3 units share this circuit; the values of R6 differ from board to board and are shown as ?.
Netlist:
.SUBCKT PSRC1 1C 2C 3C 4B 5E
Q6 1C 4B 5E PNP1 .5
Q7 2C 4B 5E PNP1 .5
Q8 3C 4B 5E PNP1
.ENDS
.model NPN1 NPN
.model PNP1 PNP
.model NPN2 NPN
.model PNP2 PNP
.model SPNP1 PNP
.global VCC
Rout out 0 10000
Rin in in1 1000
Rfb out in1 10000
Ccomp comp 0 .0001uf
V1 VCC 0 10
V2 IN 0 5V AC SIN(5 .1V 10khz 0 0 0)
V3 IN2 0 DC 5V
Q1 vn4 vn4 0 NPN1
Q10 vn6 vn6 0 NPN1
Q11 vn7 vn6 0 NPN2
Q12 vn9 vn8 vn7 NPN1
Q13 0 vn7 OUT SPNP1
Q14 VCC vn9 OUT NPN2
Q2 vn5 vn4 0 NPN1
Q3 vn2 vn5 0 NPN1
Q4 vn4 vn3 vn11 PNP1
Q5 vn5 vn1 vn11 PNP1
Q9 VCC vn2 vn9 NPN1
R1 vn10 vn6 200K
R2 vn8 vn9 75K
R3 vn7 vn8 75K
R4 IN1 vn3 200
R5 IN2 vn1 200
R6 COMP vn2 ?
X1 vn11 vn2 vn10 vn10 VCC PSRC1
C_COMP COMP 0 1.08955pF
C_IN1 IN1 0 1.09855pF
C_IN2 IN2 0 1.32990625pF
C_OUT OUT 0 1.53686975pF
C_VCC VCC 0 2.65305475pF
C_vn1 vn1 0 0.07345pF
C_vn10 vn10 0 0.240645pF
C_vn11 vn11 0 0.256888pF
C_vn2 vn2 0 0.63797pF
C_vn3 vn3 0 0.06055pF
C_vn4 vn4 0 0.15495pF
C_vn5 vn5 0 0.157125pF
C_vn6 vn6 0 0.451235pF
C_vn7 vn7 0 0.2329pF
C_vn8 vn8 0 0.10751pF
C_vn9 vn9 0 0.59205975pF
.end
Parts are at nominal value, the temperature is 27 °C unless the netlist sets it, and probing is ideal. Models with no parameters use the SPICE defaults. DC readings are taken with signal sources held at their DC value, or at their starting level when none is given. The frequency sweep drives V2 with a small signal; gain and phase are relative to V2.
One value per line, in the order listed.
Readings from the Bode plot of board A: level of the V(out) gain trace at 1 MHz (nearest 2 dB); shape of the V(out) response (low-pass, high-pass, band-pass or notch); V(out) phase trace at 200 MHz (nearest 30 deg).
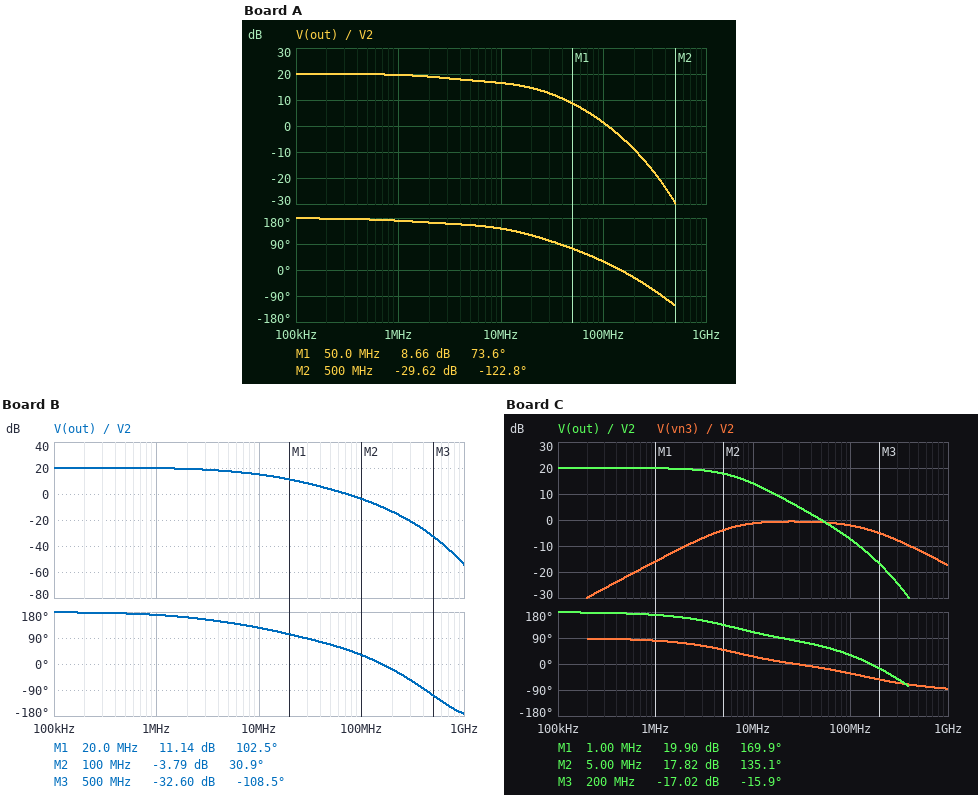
20 dB
low-pass
-30 deg
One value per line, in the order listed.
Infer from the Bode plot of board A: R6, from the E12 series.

470 Ω
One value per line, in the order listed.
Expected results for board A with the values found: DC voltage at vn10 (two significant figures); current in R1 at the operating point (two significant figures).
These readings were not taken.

9.3 V
43 µA
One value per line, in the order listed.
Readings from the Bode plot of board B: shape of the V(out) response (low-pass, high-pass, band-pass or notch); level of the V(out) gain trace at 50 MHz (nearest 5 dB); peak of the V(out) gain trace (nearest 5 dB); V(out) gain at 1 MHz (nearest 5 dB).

low-pass
5 dB
20 dB
20 dB
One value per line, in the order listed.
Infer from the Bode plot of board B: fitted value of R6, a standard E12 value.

270 Ω
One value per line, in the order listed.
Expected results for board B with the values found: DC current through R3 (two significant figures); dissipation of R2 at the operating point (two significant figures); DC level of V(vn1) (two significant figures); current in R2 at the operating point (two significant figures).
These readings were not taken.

9.1 µA
6.7 µW
5.0 V
9.5 µA
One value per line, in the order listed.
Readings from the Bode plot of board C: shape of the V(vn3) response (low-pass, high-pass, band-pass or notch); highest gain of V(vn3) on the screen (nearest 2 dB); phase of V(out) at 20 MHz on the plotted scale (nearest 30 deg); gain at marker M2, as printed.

band-pass
0 dB
90 deg
17.82 dB
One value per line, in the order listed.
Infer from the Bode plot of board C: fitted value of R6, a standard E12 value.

180 Ω
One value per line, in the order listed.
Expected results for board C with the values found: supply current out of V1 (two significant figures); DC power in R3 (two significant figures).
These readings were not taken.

630 µA
6.3 µW
